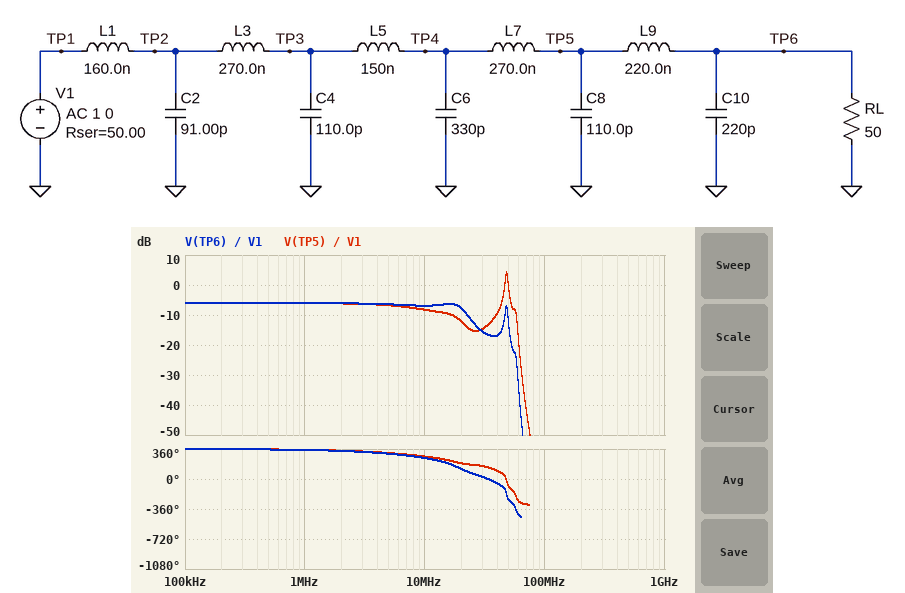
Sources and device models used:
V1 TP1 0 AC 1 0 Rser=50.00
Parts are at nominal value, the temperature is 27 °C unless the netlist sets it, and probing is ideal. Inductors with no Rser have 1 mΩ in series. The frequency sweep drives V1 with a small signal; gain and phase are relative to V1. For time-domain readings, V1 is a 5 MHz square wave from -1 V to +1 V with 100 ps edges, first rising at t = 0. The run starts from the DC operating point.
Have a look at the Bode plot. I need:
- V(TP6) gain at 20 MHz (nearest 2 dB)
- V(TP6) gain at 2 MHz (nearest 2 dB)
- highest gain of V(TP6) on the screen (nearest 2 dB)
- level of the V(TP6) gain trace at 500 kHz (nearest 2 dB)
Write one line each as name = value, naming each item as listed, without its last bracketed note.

V(TP6) gain at 20 MHz = -8 dB
V(TP6) gain at 2 MHz = -6 dB
highest gain of V(TP6) on the screen = -6 dB
level of the V(TP6) gain trace at 500 kHz = -6 dB
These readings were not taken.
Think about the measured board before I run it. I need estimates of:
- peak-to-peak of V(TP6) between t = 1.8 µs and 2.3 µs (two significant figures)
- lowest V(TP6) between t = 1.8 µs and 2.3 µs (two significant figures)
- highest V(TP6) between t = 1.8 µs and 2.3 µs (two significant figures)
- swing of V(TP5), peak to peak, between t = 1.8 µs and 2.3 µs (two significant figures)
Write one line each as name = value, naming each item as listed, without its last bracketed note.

peak-to-peak of V(TP6) between t = 1.8 µs and 2.3 µs = 1.1 V
lowest V(TP6) between t = 1.8 µs and 2.3 µs = -560 mV
highest V(TP6) between t = 1.8 µs and 2.3 µs = 560 mV
swing of V(TP5), peak to peak, between t = 1.8 µs and 2.3 µs = 1.2 V
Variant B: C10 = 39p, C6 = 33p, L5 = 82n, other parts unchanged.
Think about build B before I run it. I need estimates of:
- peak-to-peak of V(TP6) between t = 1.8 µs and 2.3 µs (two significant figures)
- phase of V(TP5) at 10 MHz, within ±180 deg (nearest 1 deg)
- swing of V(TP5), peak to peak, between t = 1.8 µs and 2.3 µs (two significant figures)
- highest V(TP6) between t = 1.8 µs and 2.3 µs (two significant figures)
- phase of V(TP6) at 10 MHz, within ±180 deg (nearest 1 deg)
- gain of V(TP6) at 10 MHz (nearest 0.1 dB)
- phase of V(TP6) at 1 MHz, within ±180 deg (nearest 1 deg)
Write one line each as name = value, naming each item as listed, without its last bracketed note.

peak-to-peak of V(TP6) between t = 1.8 µs and 2.3 µs = 1.3 V
phase of V(TP5) at 10 MHz, within ±180 deg = -55 deg
swing of V(TP5), peak to peak, between t = 1.8 µs and 2.3 µs = 1.4 V
highest V(TP6) between t = 1.8 µs and 2.3 µs = 670 mV
phase of V(TP6) at 10 MHz, within ±180 deg = -71 deg
gain of V(TP6) at 10 MHz = -6.0 dB
phase of V(TP6) at 1 MHz, within ±180 deg = -7 deg
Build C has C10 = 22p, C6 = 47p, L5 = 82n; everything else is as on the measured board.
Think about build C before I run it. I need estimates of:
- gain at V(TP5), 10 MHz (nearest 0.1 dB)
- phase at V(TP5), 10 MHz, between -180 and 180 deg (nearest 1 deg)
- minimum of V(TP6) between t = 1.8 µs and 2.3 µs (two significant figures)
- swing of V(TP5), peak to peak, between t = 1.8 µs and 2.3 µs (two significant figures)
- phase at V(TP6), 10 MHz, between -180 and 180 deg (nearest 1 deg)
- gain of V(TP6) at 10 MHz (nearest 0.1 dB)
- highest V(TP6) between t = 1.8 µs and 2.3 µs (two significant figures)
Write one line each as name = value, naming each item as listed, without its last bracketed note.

gain at V(TP5), 10 MHz = -5.9 dB
phase at V(TP5), 10 MHz, between -180 and 180 deg = -55 deg
minimum of V(TP6) between t = 1.8 µs and 2.3 µs = -660 mV
swing of V(TP5), peak to peak, between t = 1.8 µs and 2.3 µs = 1.5 V
phase at V(TP6), 10 MHz, between -180 and 180 deg = -71 deg
gain of V(TP6) at 10 MHz = -6.0 dB
highest V(TP6) between t = 1.8 µs and 2.3 µs = 660 mV
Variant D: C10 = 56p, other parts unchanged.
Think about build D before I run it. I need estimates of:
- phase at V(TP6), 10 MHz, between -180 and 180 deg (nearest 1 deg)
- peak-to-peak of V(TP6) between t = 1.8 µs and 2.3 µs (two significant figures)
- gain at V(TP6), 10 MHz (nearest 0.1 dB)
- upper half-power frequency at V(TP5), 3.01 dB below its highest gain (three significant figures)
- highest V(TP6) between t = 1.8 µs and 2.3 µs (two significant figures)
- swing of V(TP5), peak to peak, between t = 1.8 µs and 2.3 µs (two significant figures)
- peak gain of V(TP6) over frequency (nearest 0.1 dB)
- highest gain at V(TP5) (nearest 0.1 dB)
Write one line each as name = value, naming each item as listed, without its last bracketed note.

phase at V(TP6), 10 MHz, between -180 and 180 deg = -100 deg
peak-to-peak of V(TP6) between t = 1.8 µs and 2.3 µs = 1.0 V
gain at V(TP6), 10 MHz = -6.8 dB
upper half-power frequency at V(TP5), 3.01 dB below its highest gain = 22.1 MHz
highest V(TP6) between t = 1.8 µs and 2.3 µs = 520 mV
swing of V(TP5), peak to peak, between t = 1.8 µs and 2.3 µs = 1.1 V
peak gain of V(TP6) over frequency = -6.0 dB
highest gain at V(TP5) = -6.0 dB
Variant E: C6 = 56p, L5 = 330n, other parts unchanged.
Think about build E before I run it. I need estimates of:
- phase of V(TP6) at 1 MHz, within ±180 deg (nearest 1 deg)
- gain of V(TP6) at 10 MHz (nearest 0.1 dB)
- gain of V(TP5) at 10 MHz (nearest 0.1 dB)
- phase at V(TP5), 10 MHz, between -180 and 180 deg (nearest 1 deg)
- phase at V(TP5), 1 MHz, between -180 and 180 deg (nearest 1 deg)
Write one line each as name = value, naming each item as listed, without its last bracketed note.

phase of V(TP6) at 1 MHz, within ±180 deg = -10 deg
gain of V(TP6) at 10 MHz = -6.5 dB
gain of V(TP5) at 10 MHz = -7.9 dB
phase at V(TP5), 10 MHz, between -180 and 180 deg = -80 deg
phase at V(TP5), 1 MHz, between -180 and 180 deg = -8 deg
